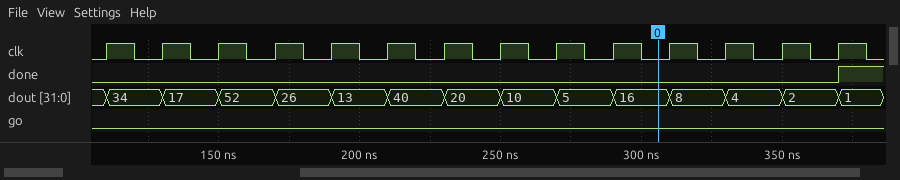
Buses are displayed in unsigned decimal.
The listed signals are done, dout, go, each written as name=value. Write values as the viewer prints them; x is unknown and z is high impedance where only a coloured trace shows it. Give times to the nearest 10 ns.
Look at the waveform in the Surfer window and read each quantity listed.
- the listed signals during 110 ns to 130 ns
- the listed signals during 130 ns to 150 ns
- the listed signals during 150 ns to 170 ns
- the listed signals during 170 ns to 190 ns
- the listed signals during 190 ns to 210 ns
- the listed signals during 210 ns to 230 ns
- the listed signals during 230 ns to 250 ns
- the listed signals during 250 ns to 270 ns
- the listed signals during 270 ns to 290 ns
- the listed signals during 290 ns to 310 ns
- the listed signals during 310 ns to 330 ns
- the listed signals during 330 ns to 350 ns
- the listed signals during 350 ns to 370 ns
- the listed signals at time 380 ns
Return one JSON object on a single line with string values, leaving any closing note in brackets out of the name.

{"the listed signals during 110 ns to 130 ns": "done=0, dout=34, go=0", "the listed signals during 130 ns to 150 ns": "done=0, dout=17, go=0", "the listed signals during 150 ns to 170 ns": "done=0, dout=52, go=0", "the listed signals during 170 ns to 190 ns": "done=0, dout=26, go=0", "the listed signals during 190 ns to 210 ns": "done=0, dout=13, go=0", "the listed signals during 210 ns to 230 ns": "done=0, dout=40, go=0", "the listed signals during 230 ns to 250 ns": "done=0, dout=20, go=0", "the listed signals during 250 ns to 270 ns": "done=0, dout=10, go=0", "the listed signals during 270 ns to 290 ns": "done=0, dout=5, go=0", "the listed signals during 290 ns to 310 ns": "done=0, dout=16, go=0", "the listed signals during 310 ns to 330 ns": "done=0, dout=8, go=0", "the listed signals during 330 ns to 350 ns": "done=0, dout=4, go=0", "the listed signals during 350 ns to 370 ns": "done=0, dout=2, go=0", "the listed signals at time 380 ns": "done=1, dout=1, go=0"}
